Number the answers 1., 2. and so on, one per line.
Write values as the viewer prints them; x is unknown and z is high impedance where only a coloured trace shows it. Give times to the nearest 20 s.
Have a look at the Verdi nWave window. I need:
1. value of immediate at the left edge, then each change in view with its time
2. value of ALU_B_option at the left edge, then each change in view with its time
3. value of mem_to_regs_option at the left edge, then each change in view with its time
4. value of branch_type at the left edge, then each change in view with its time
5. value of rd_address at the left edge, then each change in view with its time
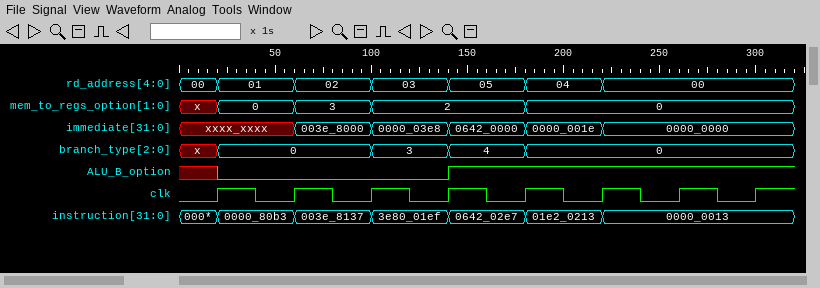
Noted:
1. xxxx_xxxx, 003e_8000 at 60 s, 0000_03e8 at 100 s, 0642_0000 at 140 s, 0000_001e at 180 s, 0000_0000 at 220 s
2. x, 0 at 20 s, 1 at 140 s
3. x, 0 at 20 s, 3 at 60 s, 2 at 100 s, 0 at 180 s
4. x, 0 at 20 s, 3 at 100 s, 4 at 140 s, 0 at 180 s
5. 00, 01 at 20 s, 02 at 60 s, 03 at 100 s, 05 at 140 s, 04 at 180 s, 00 at 220 s
